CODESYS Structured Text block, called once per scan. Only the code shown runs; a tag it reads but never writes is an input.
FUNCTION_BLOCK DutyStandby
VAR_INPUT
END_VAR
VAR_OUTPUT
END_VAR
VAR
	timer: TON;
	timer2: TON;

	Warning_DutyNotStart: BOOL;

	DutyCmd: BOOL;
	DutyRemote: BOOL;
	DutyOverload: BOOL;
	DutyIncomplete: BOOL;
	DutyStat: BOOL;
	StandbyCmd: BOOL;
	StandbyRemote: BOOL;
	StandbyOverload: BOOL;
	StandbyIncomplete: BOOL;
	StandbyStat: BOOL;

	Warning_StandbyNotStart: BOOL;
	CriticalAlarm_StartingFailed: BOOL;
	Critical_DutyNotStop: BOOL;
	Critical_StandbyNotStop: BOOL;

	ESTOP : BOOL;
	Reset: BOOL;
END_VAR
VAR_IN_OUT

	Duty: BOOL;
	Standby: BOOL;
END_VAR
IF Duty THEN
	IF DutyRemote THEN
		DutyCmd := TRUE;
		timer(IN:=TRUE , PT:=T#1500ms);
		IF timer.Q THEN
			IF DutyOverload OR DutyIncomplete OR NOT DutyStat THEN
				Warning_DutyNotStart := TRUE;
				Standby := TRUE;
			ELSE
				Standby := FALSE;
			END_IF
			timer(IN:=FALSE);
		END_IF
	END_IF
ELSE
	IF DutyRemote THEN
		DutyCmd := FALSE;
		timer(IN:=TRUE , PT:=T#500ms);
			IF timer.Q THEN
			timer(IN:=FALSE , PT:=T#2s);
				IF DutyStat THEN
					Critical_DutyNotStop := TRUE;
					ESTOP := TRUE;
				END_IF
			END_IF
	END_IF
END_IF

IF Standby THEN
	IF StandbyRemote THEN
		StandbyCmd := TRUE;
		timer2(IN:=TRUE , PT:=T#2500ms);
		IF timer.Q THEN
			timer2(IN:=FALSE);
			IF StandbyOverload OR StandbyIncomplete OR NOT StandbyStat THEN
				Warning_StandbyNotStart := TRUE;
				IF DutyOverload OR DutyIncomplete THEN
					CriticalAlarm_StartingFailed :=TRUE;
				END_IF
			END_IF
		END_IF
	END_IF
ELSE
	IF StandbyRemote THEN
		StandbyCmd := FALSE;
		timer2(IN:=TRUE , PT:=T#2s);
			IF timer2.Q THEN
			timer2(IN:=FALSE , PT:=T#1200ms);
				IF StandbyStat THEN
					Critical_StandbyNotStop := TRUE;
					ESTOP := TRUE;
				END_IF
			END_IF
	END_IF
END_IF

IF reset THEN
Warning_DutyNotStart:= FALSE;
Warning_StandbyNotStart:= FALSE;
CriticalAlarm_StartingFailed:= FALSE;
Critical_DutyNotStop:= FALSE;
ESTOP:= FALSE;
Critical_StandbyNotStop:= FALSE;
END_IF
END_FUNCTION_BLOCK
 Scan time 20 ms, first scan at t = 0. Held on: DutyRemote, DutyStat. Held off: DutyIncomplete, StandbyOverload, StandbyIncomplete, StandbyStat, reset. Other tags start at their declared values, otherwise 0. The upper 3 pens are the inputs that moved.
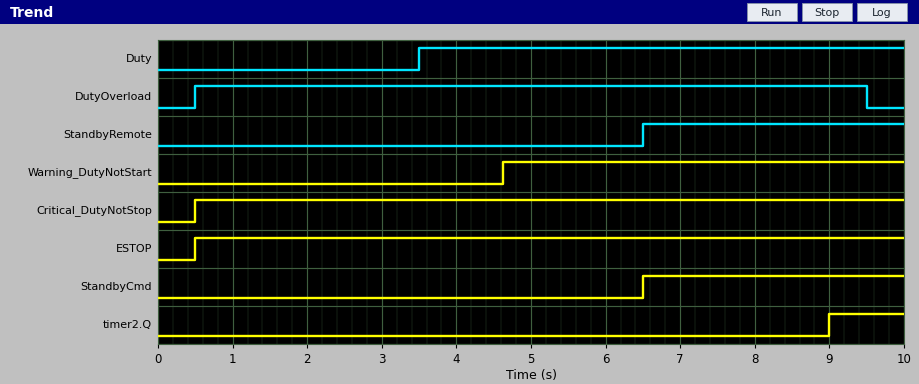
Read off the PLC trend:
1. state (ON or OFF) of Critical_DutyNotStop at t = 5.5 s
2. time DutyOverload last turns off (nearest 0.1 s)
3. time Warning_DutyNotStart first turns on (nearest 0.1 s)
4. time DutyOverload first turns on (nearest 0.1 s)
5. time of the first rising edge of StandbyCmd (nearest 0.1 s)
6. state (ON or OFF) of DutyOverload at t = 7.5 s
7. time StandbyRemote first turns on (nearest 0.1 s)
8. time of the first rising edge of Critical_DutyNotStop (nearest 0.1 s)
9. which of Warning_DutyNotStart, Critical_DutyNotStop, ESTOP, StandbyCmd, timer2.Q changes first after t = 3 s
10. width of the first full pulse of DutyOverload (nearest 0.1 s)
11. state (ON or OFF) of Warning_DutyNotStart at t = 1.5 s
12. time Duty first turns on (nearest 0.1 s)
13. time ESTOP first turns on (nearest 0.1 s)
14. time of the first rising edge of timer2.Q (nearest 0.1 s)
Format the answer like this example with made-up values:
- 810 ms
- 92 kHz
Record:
- ON
- 9.5 s
- 4.6 s
- 0.5 s
- 6.5 s
- ON
- 6.5 s
- 0.5 s
- Warning_DutyNotStart
- 9.0 s
- OFF
- 3.5 s
- 0.5 s
- 9.0 s
